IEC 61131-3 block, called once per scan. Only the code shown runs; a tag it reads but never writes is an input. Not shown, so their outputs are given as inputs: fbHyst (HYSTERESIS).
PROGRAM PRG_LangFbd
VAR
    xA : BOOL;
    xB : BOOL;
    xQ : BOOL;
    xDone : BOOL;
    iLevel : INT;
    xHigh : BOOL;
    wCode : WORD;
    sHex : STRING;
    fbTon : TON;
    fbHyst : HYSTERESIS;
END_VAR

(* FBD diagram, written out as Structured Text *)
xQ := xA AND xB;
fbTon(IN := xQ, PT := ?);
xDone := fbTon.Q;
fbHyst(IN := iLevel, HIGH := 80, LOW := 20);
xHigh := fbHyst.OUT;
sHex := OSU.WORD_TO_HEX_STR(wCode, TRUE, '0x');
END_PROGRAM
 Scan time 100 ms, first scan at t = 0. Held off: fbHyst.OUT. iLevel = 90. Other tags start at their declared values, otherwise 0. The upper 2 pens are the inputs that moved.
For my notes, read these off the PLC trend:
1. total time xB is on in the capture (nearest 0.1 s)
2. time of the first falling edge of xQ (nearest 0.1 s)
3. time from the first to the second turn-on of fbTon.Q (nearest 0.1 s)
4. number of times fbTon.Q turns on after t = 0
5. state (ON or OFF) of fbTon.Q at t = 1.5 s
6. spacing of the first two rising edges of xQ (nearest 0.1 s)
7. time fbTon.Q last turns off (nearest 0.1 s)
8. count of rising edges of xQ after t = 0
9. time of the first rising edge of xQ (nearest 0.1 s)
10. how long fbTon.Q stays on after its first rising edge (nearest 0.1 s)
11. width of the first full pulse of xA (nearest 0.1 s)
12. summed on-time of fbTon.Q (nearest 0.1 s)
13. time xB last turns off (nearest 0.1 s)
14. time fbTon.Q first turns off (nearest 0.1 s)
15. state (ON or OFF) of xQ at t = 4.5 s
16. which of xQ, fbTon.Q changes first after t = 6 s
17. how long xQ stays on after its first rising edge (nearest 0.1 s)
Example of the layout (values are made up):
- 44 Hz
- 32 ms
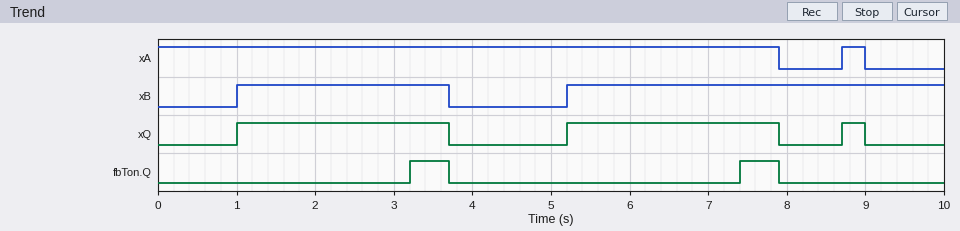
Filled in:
- 7.5 s
- 3.7 s
- 4.2 s
- 2
- OFF
- 4.2 s
- 7.9 s
- 3
- 1.0 s
- 0.5 s
- 0.3 s
- 1.0 s
- 3.7 s
- 3.7 s
- OFF
- fbTon.Q
- 2.7 s
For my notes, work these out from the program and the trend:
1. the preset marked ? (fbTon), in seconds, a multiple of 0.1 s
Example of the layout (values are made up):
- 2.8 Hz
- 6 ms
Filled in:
- 2.2 s
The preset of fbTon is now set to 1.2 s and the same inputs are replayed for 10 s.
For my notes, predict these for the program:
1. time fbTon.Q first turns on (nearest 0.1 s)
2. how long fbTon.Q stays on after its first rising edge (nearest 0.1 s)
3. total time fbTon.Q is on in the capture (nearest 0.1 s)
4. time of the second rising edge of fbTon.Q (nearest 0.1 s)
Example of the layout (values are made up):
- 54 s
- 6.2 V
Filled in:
- 2.2 s
- 1.5 s
- 3.0 s
- 6.4 s
